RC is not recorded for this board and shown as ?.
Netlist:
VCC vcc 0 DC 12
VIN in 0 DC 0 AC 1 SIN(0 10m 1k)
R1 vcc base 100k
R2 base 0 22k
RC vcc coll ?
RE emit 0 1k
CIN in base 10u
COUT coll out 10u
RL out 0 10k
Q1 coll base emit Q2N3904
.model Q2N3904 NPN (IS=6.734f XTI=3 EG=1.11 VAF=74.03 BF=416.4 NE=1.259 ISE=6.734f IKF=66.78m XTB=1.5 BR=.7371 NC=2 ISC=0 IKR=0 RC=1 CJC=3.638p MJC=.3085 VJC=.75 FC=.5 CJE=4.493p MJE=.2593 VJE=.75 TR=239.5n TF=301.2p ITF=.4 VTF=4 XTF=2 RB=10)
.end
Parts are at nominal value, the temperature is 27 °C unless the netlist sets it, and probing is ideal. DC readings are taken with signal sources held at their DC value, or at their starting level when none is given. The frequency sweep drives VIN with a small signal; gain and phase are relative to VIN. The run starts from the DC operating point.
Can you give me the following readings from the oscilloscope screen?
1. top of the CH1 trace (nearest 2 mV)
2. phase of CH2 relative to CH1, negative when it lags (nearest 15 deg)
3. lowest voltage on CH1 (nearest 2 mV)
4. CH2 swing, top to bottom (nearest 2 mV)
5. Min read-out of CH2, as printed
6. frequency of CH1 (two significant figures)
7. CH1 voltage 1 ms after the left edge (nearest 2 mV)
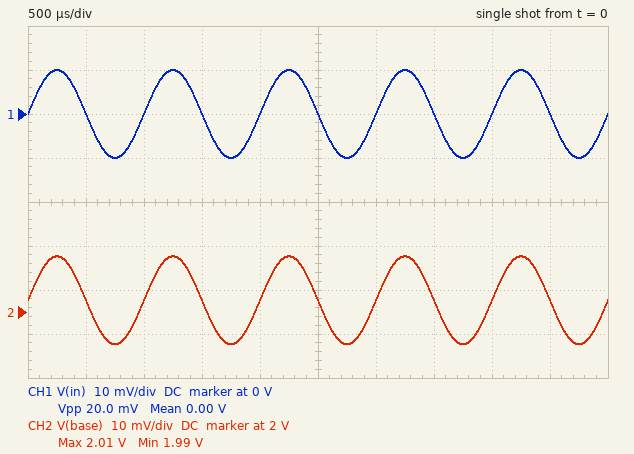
10 mV
0 deg
-10 mV
20 mV
1.99 V
1.0 kHz
0 V
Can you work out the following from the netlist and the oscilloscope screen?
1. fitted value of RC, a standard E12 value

2.7 kΩ
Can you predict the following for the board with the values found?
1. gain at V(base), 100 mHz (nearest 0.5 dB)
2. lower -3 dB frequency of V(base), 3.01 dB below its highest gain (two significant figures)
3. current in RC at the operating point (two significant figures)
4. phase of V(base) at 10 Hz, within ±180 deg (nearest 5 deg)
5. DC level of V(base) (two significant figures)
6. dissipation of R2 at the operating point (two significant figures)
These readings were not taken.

-20.0 dB
980 mHz
1.3 mA
5 deg
2.0 V
180 µW
